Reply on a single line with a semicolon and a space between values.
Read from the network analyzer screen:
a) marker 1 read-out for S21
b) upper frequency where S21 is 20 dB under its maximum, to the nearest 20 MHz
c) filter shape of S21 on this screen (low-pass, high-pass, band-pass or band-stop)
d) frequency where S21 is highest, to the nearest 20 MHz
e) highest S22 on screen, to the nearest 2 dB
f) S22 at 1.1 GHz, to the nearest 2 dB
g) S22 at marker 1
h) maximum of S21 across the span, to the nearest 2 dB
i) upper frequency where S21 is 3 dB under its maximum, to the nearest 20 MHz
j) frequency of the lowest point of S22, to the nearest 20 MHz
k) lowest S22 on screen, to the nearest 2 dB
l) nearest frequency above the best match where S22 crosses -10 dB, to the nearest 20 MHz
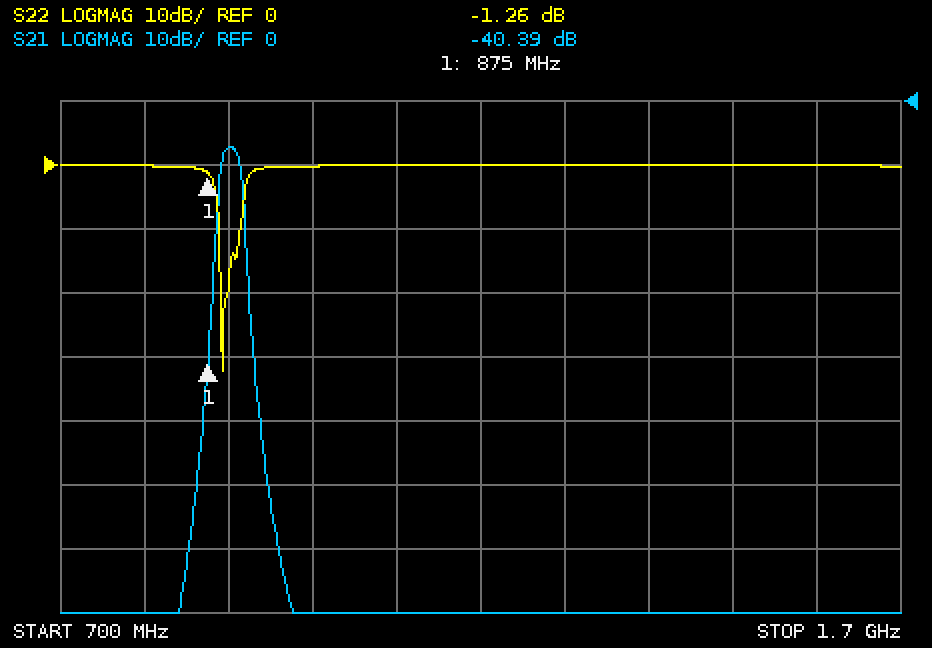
-40.39 dB; 920 MHz; band-pass; 900 MHz; 0 dB; 0 dB; -1.26 dB; -8 dB; 920 MHz; 900 MHz; -32 dB; 920 MHz
